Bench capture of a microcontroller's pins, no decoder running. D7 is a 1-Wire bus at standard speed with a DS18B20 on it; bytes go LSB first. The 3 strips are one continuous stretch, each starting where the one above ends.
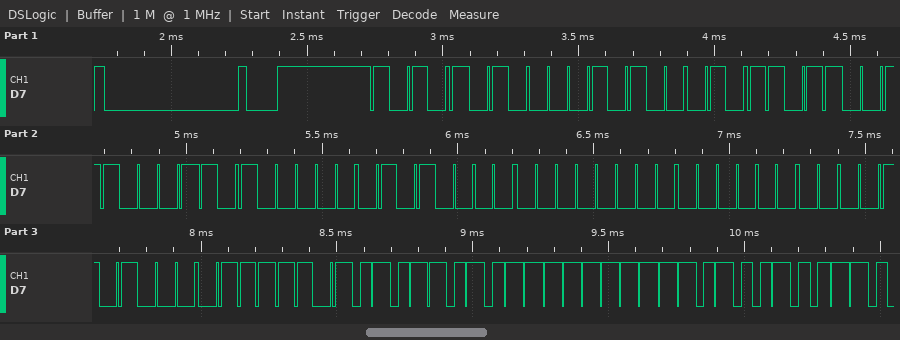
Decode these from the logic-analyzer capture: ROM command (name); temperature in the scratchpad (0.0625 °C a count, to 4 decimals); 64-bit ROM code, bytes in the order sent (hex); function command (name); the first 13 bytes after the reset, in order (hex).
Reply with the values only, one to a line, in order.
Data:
Match ROM
-10.3750 °C
28 DA 8C 05 0A 00 00 14
Read Scratchpad
55 28 DA 8C 05 0A 00 00 14 BE 5A FF 4B
